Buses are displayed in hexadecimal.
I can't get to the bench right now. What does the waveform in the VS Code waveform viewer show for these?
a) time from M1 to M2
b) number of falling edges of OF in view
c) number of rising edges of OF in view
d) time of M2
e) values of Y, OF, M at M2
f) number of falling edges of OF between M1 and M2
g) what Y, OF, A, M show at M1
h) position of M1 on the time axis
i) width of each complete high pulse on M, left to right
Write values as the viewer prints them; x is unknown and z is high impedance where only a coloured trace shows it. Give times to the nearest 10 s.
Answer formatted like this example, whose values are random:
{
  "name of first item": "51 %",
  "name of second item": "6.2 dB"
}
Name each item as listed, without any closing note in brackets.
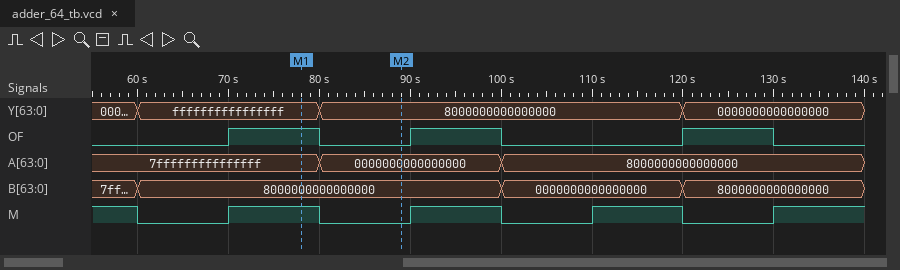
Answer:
{
  "time from M1 to M2": "10 s",
  "number of falling edges of OF in view": "3",
  "number of rising edges of OF in view": "3",
  "time of M2": "90 s",
  "values of Y, OF, M at M2": "Y=8000000000000000, OF=0, M=0",
  "number of falling edges of OF between M1 and M2": "1",
  "what Y, OF, A, M show at M1": "Y=ffffffffffffffff, OF=1, A=7fffffffffffffff, M=1",
  "position of M1 on the time axis": "80 s",
  "width of each complete high pulse on M, left to right": "10 s, 10 s, 10 s"
}
